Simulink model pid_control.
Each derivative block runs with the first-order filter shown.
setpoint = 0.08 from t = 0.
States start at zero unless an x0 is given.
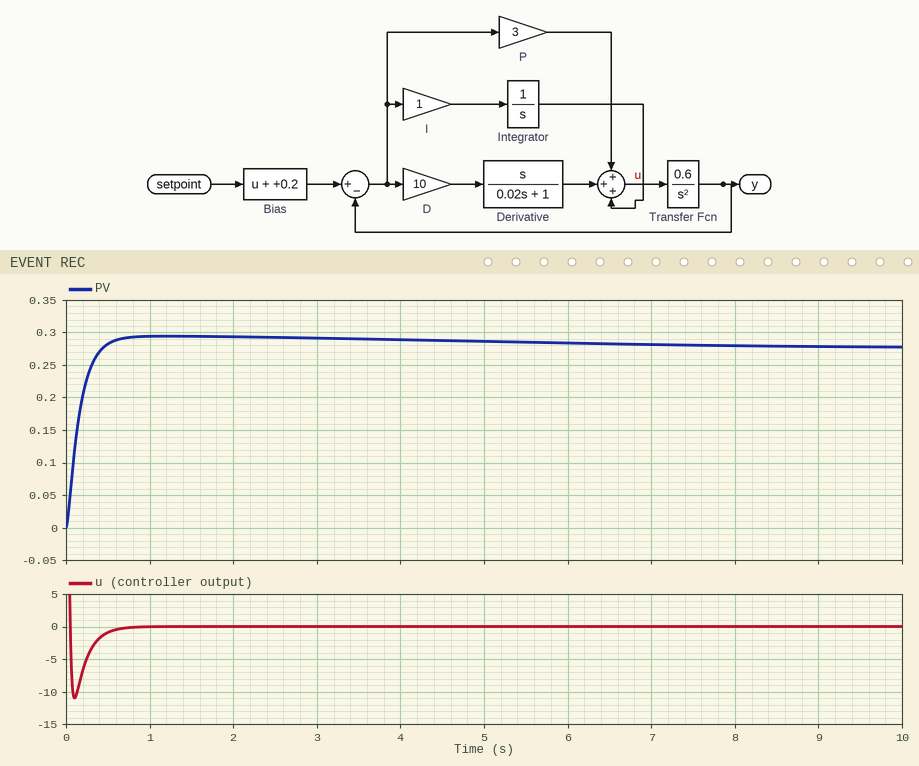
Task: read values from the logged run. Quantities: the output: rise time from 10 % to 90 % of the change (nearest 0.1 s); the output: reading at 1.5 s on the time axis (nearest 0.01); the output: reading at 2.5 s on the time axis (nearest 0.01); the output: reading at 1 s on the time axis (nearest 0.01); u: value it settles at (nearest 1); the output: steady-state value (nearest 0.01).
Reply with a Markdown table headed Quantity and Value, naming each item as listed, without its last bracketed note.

| Quantity | Value |
|---|---|
| the output: rise time from 10 % to 90 % of the change | 0.3 s |
| the output: reading at 1.5 s on the time axis | 0.29 |
| the output: reading at 2.5 s on the time axis | 0.29 |
| the output: reading at 1 s on the time axis | 0.29 |
| u: value it settles at | 0 |
| the output: steady-state value | 0.28 |
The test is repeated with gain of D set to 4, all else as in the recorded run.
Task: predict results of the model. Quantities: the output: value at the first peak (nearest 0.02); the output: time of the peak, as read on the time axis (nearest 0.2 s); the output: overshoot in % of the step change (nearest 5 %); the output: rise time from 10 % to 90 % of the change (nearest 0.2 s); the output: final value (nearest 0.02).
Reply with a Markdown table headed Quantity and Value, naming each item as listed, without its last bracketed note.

| Quantity | Value |
|---|---|
| the output: value at the first peak | 0.34 |
| the output: time of the peak, as read on the time axis | 1.6 s |
| the output: overshoot in % of the step change | 20 % |
| the output: rise time from 10 % to 90 % of the change | 0.6 s |
| the output: final value | 0.28 |
